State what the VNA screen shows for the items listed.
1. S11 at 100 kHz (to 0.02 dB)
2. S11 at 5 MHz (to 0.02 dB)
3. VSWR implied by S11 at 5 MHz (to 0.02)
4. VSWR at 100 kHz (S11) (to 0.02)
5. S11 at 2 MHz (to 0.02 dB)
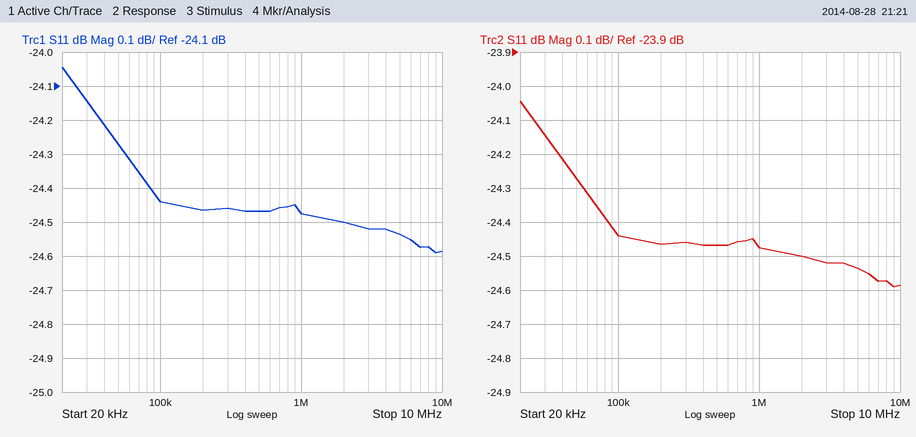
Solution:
-24.44 dB
-24.54 dB
1.12
1.12
-24.50 dB
